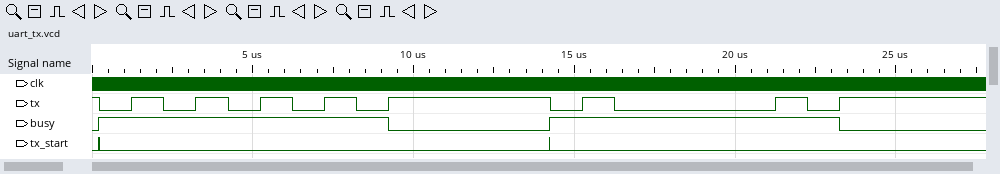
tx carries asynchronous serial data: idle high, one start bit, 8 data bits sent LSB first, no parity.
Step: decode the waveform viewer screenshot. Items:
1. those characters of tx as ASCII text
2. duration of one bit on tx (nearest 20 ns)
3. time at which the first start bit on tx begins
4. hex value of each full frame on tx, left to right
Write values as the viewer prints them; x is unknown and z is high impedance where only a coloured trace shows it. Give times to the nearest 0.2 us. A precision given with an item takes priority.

"UA"
1000 ns
0 us
55, 41
